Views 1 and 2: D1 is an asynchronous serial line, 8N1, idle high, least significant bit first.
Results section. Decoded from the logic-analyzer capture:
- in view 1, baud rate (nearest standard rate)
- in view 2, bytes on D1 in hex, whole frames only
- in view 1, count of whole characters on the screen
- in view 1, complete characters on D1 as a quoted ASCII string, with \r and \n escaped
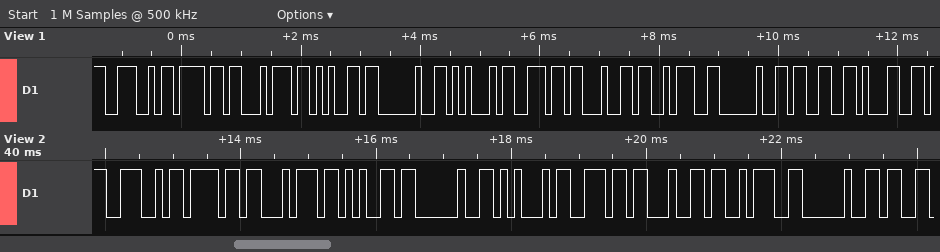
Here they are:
9600 baud
0x4E 0x6F 0x74 0x65 0x20 0x45 0x6E 0x64 0x3A 0x20
12
"Note End: 31"
